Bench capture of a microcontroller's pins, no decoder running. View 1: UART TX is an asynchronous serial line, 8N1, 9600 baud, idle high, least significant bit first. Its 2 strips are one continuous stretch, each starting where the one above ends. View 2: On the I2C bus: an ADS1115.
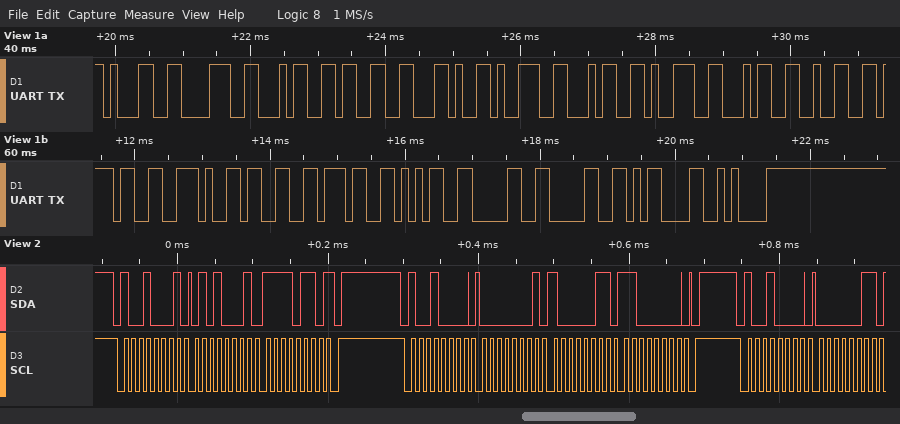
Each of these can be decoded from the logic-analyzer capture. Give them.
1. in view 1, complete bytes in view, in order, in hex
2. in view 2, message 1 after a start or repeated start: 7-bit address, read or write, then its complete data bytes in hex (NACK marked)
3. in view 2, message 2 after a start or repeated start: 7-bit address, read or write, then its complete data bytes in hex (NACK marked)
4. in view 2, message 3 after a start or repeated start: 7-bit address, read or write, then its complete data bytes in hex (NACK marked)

31 38 34 33 2C 39 34 39 34 32 37 2E 33 37 35 30 30 0D 0A
0x48 read: 51 F6 NACK
0x48 write: 01 83 C0
0x48 write: 03
